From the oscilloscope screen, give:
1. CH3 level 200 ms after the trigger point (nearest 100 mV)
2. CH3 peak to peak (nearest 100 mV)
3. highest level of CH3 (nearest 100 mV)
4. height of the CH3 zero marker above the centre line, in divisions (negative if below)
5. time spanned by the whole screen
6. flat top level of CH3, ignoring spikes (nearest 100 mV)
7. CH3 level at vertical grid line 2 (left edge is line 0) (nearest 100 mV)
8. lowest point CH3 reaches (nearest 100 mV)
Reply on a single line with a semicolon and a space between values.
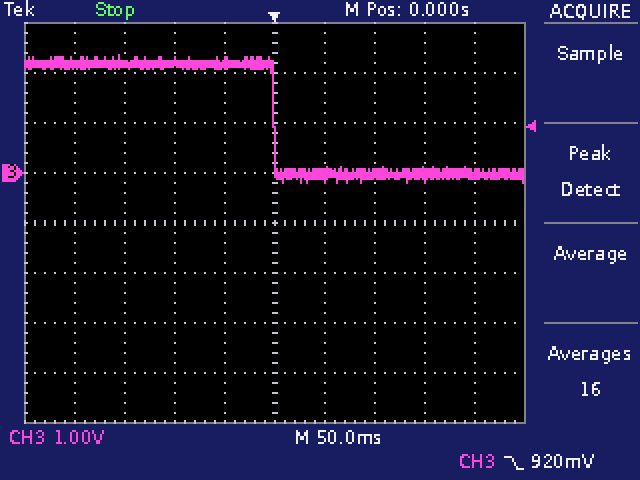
0.0 V; 2.6 V; 2.4 V; +1.0 div; 500 ms; 2.2 V; 2.2 V; -200 mV
